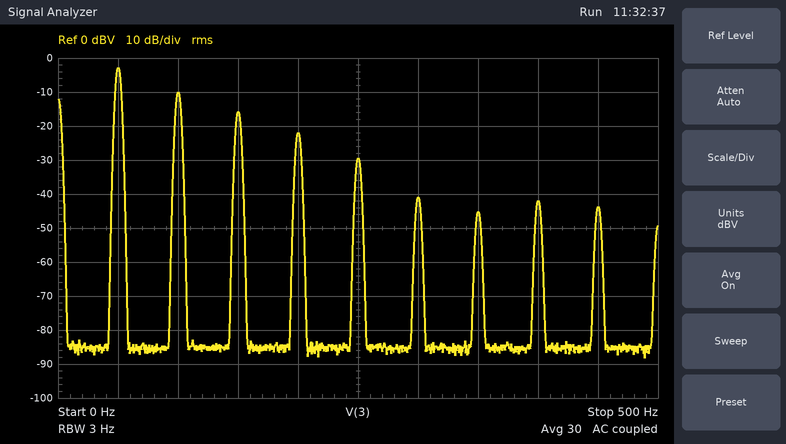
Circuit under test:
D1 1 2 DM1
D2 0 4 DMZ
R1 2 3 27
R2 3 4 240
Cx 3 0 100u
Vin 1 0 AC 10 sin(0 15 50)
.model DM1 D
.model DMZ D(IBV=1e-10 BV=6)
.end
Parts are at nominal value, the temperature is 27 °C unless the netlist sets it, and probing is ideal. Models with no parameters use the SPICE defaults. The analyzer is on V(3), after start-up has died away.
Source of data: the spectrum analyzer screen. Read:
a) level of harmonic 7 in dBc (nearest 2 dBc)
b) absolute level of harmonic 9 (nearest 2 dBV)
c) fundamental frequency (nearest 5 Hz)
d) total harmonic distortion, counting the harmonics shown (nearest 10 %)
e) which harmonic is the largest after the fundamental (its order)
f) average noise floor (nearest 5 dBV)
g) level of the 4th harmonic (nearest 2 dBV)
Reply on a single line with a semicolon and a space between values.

-42 dBc; -44 dBV; 50 Hz; 50 %; 2; -85 dBV; -22 dBV
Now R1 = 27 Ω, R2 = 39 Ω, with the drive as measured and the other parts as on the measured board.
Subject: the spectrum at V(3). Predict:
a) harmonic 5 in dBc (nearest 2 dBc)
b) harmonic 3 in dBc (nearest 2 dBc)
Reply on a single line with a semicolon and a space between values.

-40 dBc; -14 dBc
